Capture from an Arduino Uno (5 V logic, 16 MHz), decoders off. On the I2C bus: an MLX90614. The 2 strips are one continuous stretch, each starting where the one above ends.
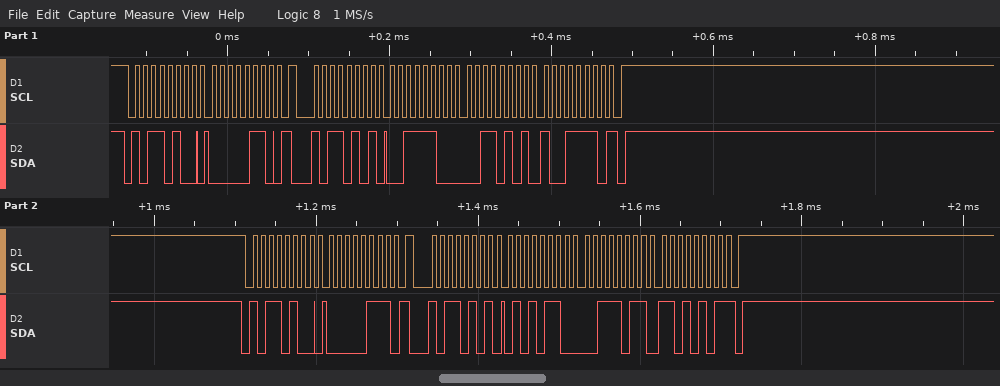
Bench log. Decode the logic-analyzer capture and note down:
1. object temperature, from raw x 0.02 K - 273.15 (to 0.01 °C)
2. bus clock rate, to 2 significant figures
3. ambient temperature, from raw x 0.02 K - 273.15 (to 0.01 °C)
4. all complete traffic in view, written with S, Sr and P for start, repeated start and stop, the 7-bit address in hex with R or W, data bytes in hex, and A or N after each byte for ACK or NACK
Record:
30.65 °C
100 kHz
-0.59 °C
S 5AW A 06 A Sr 5AR A 3C A 35 A 9E N P S 5AW A 07 A Sr 5AR A 56 A 3B A D5 N P
